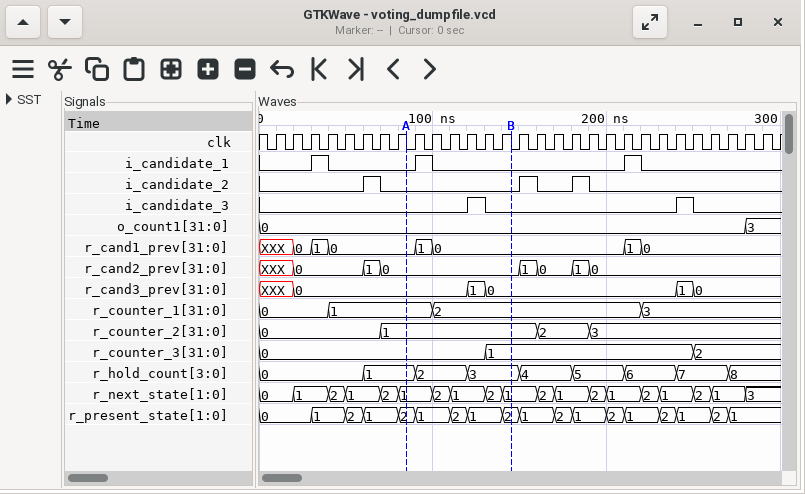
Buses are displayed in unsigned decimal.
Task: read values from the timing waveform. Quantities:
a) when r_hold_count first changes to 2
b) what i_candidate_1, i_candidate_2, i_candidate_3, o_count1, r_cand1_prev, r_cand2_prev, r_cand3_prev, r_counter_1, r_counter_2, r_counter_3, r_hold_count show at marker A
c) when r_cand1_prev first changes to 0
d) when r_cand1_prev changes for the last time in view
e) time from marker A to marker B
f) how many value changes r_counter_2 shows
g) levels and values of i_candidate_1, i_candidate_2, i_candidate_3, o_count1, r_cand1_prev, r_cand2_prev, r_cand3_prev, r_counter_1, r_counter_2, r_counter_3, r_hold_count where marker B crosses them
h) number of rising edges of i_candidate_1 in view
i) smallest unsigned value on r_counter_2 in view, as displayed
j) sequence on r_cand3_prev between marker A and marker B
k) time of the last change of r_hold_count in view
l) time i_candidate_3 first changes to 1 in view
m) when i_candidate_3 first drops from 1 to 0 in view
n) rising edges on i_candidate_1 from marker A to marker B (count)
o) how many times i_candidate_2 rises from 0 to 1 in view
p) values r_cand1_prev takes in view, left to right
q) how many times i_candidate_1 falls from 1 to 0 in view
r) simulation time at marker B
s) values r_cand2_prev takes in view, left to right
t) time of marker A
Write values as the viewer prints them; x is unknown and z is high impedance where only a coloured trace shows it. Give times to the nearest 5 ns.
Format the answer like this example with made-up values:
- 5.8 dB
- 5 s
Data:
- 90 ns
- i_candidate_1=0, i_candidate_2=0, i_candidate_3=0, o_count1=0, r_cand1_prev=0, r_cand2_prev=0, r_cand3_prev=0, r_counter_1=1, r_counter_2=1, r_counter_3=0, r_hold_count=1
- 20 ns
- 220 ns
- 60 ns
- 3
- i_candidate_1=0, i_candidate_2=0, i_candidate_3=0, o_count1=0, r_cand1_prev=0, r_cand2_prev=0, r_cand3_prev=0, r_counter_1=2, r_counter_2=1, r_counter_3=1, r_hold_count=3
- 3
- 0
- 0, 1, 0
- 270 ns
- 120 ns
- 130 ns
- 1
- 3
- XXX, 0, 1, 0, 1, 0, 1, 0
- 3
- 145 ns
- XXX, 0, 1, 0, 1, 0, 1, 0
- 85 ns
